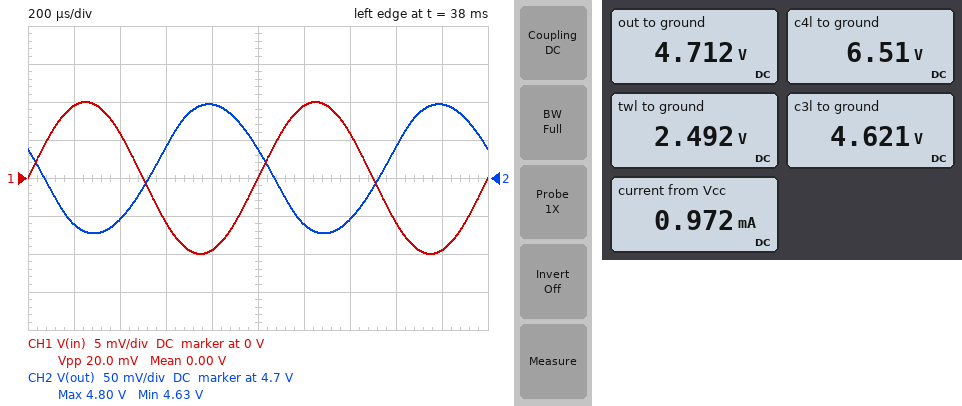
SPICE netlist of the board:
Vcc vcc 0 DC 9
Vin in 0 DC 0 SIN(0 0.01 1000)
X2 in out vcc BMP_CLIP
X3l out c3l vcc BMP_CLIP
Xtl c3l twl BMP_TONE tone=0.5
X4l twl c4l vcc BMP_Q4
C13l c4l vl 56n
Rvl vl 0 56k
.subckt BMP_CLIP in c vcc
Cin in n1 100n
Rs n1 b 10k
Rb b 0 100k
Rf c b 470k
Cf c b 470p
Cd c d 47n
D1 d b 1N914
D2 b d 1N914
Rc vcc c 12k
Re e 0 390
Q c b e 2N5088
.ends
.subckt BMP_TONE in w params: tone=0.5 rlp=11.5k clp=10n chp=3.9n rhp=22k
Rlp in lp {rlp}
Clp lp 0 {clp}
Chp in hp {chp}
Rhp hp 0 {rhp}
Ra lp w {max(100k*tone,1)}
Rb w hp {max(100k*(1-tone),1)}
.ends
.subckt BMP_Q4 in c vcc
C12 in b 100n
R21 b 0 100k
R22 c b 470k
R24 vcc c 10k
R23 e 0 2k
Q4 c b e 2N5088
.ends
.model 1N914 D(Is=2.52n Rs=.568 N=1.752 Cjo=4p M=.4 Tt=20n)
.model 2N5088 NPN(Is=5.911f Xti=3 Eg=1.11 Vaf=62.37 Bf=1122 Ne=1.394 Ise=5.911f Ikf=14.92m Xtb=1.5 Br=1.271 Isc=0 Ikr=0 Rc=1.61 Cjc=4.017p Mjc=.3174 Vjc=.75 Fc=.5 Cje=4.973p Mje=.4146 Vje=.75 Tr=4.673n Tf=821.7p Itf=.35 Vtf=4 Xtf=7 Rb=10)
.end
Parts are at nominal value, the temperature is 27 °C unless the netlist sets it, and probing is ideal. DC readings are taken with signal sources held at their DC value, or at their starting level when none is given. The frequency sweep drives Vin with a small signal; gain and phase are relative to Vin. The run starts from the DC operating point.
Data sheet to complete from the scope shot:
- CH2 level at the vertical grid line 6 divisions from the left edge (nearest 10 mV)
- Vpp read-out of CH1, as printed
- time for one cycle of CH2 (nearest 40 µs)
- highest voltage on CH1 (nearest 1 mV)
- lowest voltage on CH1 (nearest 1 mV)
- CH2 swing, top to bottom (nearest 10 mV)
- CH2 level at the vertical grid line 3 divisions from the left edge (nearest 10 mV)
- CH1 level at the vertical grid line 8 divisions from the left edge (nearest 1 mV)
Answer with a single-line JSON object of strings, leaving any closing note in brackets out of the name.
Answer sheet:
{"CH2 level at the vertical grid line 6 divisions from the left edge": "4.64 V", "Vpp read-out of CH1, as printed": "20.0 mV", "time for one cycle of CH2": "1.00 ms", "highest voltage on CH1": "10 mV", "lowest voltage on CH1": "-10 mV", "CH2 swing, top to bottom": "170 mV", "CH2 level at the vertical grid line 3 divisions from the left edge": "4.74 V", "CH1 level at the vertical grid line 8 divisions from the left edge": "-6 mV"}
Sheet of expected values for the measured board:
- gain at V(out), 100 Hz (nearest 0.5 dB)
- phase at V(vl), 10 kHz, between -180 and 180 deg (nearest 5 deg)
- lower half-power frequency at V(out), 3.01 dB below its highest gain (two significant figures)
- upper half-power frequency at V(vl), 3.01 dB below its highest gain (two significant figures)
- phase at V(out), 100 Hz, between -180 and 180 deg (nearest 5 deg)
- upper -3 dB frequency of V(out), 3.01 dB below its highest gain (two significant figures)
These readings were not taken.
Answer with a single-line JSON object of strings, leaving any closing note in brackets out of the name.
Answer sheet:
{"gain at V(out), 100 Hz": "20.0 dB", "phase at V(vl), 10 kHz, between -180 and 180 deg": "45 deg", "lower half-power frequency at V(out), 3.01 dB below its highest gain": "42 Hz", "upper half-power frequency at V(vl), 3.01 dB below its highest gain": "810 Hz", "phase at V(out), 100 Hz, between -180 and 180 deg": "-160 deg", "upper -3 dB frequency of V(out), 3.01 dB below its highest gain": "2.3 kHz"}
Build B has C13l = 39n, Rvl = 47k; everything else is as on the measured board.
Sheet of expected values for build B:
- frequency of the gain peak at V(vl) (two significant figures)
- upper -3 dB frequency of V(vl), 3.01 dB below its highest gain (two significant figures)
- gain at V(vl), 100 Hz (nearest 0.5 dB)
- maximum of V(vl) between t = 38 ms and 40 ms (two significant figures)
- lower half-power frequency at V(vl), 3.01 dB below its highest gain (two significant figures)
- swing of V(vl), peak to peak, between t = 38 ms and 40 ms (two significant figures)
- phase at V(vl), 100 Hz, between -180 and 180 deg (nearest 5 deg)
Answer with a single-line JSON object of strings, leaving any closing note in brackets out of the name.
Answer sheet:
{"frequency of the gain peak at V(vl)": "270 Hz", "upper -3 dB frequency of V(vl), 3.01 dB below its highest gain": "830 Hz", "gain at V(vl), 100 Hz": "40.5 dB", "maximum of V(vl) between t = 38 ms and 40 ms": "340 mV", "lower half-power frequency at V(vl), 3.01 dB below its highest gain": "96 Hz", "swing of V(vl), peak to peak, between t = 38 ms and 40 ms": "690 mV", "phase at V(vl), 100 Hz, between -180 and 180 deg": "-85 deg"}
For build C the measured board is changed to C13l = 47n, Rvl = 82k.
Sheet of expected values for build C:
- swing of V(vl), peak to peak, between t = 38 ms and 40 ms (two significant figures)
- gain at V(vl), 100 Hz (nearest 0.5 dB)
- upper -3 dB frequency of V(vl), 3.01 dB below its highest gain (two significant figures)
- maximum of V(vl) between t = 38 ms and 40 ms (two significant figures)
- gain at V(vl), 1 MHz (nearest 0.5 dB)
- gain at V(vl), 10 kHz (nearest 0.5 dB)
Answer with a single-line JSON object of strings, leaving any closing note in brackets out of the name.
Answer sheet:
{"swing of V(vl), peak to peak, between t = 38 ms and 40 ms": "740 mV", "gain at V(vl), 100 Hz": "42.5 dB", "upper -3 dB frequency of V(vl), 3.01 dB below its highest gain": "800 Hz", "maximum of V(vl) between t = 38 ms and 40 ms": "370 mV", "gain at V(vl), 1 MHz": "-53.5 dB", "gain at V(vl), 10 kHz": "19.0 dB"}
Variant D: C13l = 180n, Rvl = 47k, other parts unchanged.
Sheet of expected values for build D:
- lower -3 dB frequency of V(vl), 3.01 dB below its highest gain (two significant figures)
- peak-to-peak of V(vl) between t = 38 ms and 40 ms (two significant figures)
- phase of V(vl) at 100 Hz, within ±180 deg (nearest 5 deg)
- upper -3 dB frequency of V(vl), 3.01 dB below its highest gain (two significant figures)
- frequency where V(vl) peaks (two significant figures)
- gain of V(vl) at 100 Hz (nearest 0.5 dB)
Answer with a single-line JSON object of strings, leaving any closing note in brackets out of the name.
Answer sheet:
{"lower -3 dB frequency of V(vl), 3.01 dB below its highest gain": "72 Hz", "peak-to-peak of V(vl) between t = 38 ms and 40 ms": "700 mV", "phase of V(vl) at 100 Hz, within ±180 deg": "-115 deg", "upper -3 dB frequency of V(vl), 3.01 dB below its highest gain": "790 Hz", "frequency where V(vl) peaks": "230 Hz", "gain of V(vl) at 100 Hz": "42.5 dB"}
